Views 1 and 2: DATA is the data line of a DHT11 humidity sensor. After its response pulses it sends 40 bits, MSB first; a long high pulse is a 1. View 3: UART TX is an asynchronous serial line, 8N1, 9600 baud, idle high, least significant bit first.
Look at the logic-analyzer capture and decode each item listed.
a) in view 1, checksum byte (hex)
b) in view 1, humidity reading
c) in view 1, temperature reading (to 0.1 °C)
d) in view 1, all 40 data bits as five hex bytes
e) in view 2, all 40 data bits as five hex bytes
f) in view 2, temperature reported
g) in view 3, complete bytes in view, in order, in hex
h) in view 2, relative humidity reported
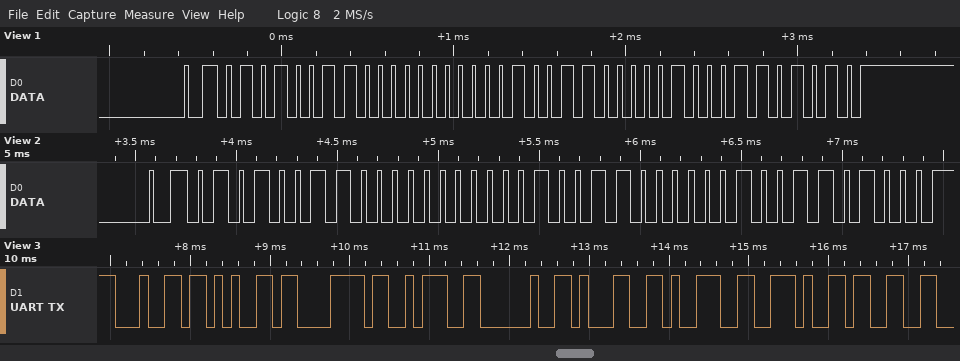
0x6A
83 %
19.4 °C
53 00 13 04 6A
53 00 13 02 68
19.2 °C
0x64 0x65 0x78 0x3A 0x20 0x31 0x39 0x2E 0x33
83 %
